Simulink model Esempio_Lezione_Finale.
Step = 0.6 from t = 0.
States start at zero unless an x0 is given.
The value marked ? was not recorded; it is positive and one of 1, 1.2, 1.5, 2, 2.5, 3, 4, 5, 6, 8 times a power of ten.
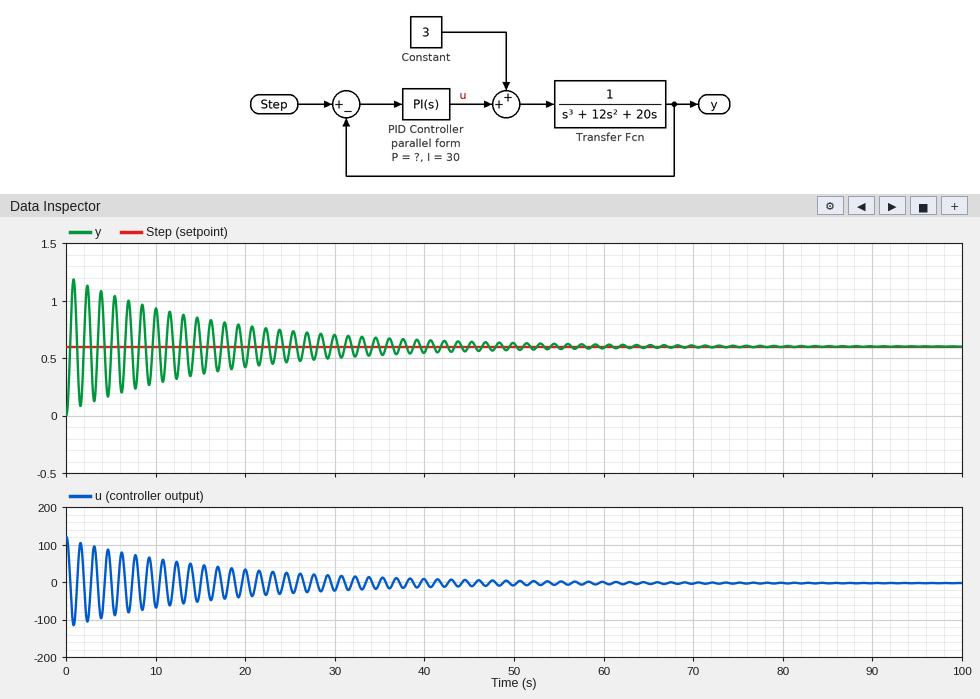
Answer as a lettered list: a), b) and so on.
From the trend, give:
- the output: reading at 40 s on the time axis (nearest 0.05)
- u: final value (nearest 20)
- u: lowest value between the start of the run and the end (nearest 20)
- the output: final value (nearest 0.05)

a) 0.55
b) 0
c) -120
d) 0.60
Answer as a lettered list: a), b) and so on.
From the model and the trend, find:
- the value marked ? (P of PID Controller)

a) 200
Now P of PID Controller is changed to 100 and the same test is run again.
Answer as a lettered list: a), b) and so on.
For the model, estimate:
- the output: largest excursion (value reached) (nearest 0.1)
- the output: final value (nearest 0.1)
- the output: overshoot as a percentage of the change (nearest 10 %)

a) 1.1
b) 0.6
c) 80 %
